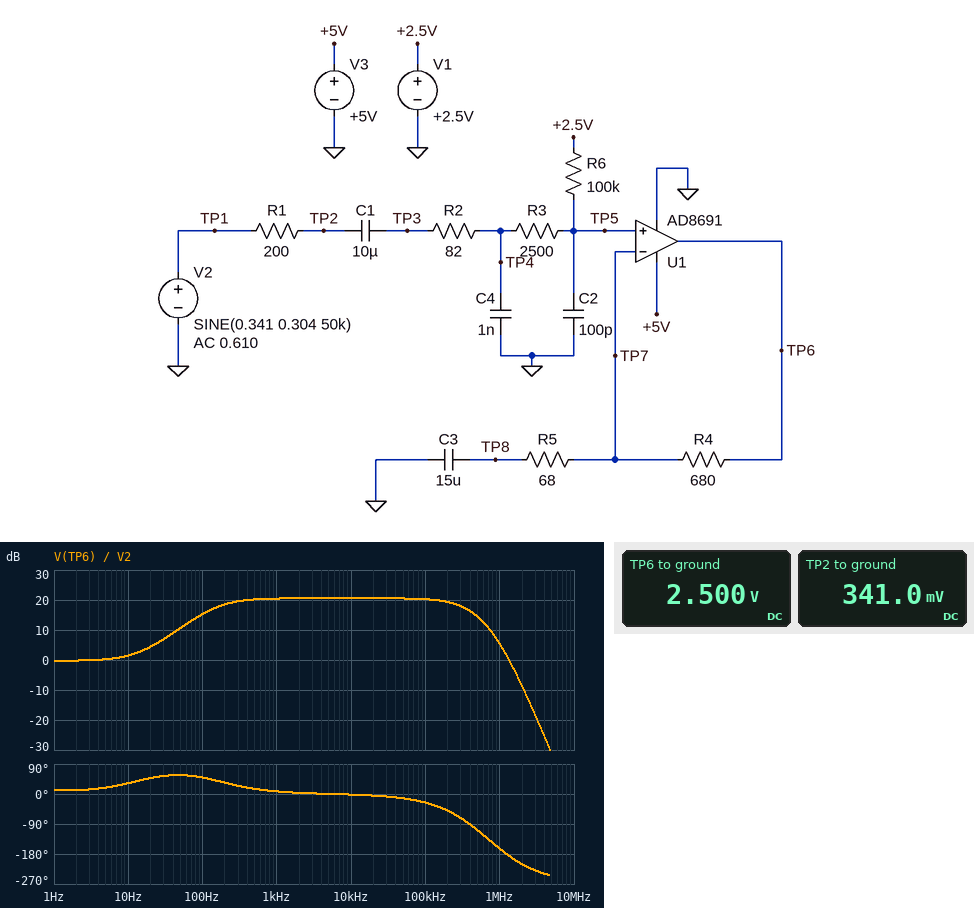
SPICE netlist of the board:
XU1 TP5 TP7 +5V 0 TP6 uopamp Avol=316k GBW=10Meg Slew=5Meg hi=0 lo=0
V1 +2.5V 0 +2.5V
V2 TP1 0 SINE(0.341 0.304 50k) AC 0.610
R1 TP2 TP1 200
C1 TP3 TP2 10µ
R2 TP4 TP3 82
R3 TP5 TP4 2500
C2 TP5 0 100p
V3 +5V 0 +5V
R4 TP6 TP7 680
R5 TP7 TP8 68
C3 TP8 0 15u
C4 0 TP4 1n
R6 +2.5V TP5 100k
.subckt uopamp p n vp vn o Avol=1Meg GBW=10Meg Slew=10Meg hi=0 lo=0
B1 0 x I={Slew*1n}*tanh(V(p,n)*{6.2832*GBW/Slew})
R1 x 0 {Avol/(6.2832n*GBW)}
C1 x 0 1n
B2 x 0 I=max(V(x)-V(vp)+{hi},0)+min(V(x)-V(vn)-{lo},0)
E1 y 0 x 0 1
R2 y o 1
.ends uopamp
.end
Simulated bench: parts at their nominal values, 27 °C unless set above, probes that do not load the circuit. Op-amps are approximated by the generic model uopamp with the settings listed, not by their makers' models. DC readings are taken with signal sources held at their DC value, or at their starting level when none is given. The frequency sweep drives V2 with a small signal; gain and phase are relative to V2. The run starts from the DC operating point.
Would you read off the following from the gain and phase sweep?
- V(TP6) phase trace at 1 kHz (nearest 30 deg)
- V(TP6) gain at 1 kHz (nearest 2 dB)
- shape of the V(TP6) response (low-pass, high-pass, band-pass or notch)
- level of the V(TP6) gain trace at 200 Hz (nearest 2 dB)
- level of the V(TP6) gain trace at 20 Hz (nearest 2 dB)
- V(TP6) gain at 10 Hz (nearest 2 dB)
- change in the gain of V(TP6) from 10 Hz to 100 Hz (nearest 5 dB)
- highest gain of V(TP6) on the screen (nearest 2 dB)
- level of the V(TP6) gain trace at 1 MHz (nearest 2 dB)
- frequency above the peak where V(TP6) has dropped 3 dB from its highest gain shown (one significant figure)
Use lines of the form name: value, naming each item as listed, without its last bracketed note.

V(TP6) phase trace at 1 kHz: 0 deg
V(TP6) gain at 1 kHz: 20 dB
shape of the V(TP6) response: band-pass
level of the V(TP6) gain trace at 200 Hz: 18 dB
level of the V(TP6) gain trace at 20 Hz: 4 dB
V(TP6) gain at 10 Hz: 2 dB
change in the gain of V(TP6) from 10 Hz to 100 Hz: 15 dB
highest gain of V(TP6) on the screen: 20 dB
level of the V(TP6) gain trace at 1 MHz: 6 dB
frequency above the peak where V(TP6) has dropped 3 dB from its highest gain shown: 300 kHz
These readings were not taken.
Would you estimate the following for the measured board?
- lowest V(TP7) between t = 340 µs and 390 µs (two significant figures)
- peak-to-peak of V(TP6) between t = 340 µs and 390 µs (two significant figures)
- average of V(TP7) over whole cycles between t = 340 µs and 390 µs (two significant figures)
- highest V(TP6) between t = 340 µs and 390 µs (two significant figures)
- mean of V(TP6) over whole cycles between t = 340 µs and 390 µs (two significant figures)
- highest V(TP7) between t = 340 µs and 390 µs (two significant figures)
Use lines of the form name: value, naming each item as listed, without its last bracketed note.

lowest V(TP7) between t = 340 µs and 390 µs: 2.3 V
peak-to-peak of V(TP6) between t = 340 µs and 390 µs: 5.0 V
average of V(TP7) over whole cycles between t = 340 µs and 390 µs: 2.5 V
highest V(TP6) between t = 340 µs and 390 µs: 5.0 V
mean of V(TP6) over whole cycles between t = 340 µs and 390 µs: 2.5 V
highest V(TP7) between t = 340 µs and 390 µs: 2.7 V
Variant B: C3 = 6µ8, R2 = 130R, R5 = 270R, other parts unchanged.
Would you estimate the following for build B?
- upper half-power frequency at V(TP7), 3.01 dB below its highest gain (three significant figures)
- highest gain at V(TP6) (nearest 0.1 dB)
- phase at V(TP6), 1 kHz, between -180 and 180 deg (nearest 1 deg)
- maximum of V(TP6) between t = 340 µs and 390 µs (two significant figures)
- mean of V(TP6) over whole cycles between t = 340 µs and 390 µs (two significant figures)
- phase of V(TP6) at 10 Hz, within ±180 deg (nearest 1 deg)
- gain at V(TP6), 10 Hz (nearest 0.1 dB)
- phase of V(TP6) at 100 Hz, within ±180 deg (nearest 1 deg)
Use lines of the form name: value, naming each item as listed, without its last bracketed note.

upper half-power frequency at V(TP7), 3.01 dB below its highest gain: 326 kHz
highest gain at V(TP6): 10.7 dB
phase at V(TP6), 1 kHz, between -180 and 180 deg: 3 deg
maximum of V(TP6) between t = 340 µs and 390 µs: 3.5 V
mean of V(TP6) over whole cycles between t = 340 µs and 390 µs: 2.5 V
phase of V(TP6) at 10 Hz, within ±180 deg: 16 deg
gain at V(TP6), 10 Hz: 0.4 dB
phase of V(TP6) at 100 Hz, within ±180 deg: 27 deg
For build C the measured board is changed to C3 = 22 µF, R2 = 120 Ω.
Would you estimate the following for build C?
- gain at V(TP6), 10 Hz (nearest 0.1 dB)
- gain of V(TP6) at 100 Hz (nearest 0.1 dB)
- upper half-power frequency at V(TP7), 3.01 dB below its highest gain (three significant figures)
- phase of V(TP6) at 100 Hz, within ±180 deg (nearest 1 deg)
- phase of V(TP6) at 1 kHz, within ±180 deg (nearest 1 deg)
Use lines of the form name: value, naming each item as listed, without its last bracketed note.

gain at V(TP6), 10 Hz: 2.9 dB
gain of V(TP6) at 100 Hz: 17.3 dB
upper half-power frequency at V(TP7), 3.01 dB below its highest gain: 304 kHz
phase of V(TP6) at 100 Hz, within ±180 deg: 41 deg
phase of V(TP6) at 1 kHz, within ±180 deg: 5 deg
